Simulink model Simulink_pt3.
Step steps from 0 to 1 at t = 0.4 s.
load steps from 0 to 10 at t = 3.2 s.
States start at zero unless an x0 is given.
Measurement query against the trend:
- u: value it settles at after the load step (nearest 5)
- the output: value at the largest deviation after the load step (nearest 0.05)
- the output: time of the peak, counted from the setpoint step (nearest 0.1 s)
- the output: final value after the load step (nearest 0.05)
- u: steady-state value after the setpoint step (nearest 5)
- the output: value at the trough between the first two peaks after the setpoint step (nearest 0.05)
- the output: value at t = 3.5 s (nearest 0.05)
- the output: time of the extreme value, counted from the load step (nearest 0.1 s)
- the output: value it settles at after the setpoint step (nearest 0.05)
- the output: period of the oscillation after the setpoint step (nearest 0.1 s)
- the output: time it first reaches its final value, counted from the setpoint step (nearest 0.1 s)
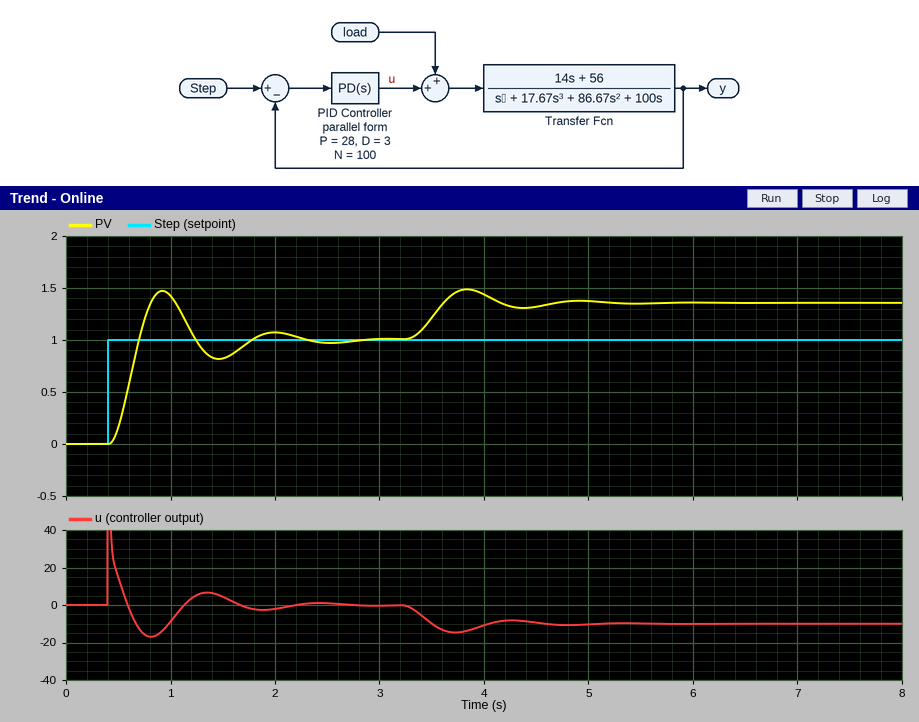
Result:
-10
1.50
0.5 s
1.35
0
0.80
1.20
0.6 s
1.00
1.1 s
0.3 s
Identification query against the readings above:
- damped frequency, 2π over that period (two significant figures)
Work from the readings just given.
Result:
5.7 rad/s
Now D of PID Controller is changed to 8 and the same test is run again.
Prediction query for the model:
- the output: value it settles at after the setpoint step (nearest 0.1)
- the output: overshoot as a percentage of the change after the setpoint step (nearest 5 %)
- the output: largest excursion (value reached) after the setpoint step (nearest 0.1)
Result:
1.0
25 %
1.3
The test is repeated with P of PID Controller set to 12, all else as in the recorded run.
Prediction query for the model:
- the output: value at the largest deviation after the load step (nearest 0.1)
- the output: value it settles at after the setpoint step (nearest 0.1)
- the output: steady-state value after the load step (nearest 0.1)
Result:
1.9
1.0
1.8
